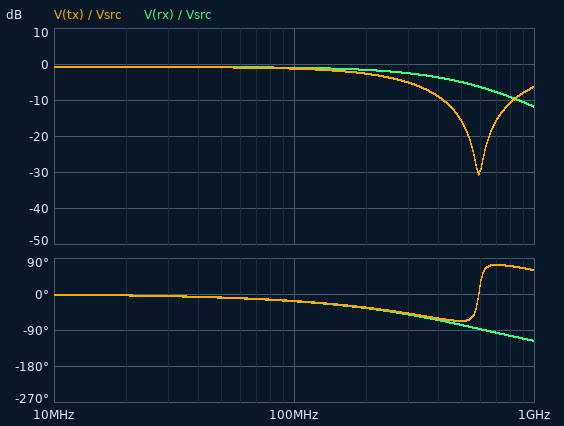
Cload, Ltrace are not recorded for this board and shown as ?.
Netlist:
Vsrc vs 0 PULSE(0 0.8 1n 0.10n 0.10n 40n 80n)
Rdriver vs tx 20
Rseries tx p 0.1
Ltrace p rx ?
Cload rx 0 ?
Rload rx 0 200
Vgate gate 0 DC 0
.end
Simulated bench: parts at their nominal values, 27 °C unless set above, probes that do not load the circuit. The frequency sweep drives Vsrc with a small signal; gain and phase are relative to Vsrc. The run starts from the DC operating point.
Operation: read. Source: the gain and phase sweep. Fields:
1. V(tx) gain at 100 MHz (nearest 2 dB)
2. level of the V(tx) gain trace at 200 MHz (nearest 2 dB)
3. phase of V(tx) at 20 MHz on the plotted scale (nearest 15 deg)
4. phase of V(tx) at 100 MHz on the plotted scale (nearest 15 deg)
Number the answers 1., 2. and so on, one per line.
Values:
1. -2 dB
2. -2 dB
3. 0 deg
4. -15 deg
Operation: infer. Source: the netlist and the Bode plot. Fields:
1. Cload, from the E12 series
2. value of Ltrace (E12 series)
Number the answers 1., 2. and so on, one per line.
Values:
1. 27 pF
2. 2.7 nH
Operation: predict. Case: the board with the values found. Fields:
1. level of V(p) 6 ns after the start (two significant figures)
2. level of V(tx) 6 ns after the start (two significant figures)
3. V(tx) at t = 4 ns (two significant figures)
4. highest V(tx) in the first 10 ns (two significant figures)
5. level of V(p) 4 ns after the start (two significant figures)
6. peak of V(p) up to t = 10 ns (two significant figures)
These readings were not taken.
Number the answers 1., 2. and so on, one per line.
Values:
1. 730 mV
2. 730 mV
3. 730 mV
4. 730 mV
5. 730 mV
6. 730 mV
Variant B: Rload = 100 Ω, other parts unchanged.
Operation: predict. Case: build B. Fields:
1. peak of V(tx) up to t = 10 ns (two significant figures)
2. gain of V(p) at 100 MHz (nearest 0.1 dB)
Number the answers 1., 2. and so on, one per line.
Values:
1. 670 mV
2. -2.0 dB
